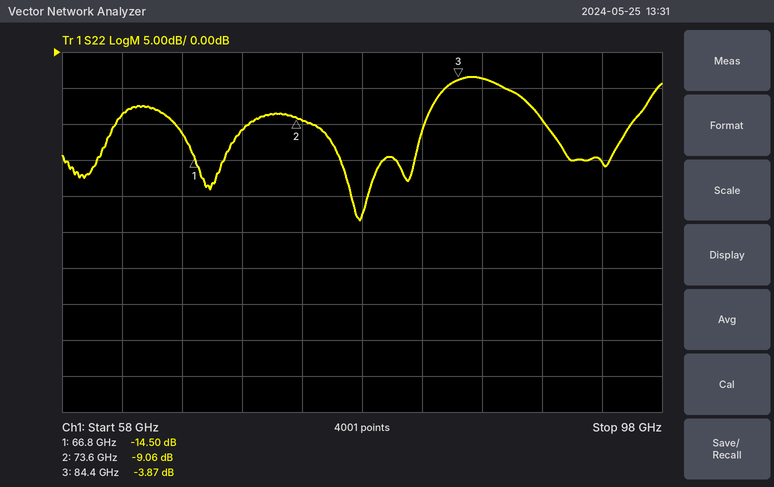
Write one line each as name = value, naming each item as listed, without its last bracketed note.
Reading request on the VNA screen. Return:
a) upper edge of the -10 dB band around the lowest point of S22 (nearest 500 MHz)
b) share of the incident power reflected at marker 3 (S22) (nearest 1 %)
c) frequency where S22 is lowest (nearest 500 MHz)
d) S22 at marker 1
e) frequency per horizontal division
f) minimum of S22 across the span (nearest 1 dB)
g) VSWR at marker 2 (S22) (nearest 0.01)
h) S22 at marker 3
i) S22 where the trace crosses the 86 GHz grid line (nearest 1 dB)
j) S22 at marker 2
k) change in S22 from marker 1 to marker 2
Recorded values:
upper edge of the -10 dB band around the lowest point of S22 = 82.0 GHz
share of the incident power reflected at marker 3 (S22) = 41 %
frequency where S22 is lowest = 78.0 GHz
S22 at marker 1 = -14.50 dB
frequency per horizontal division = 4 GHz
minimum of S22 across the span = -23 dB
VSWR at marker 2 (S22) = 2.09
S22 at marker 3 = -3.87 dB
S22 where the trace crosses the 86 GHz grid line = -4 dB
S22 at marker 2 = -9.06 dB
change in S22 from marker 1 to marker 2 = 5.44 dB
